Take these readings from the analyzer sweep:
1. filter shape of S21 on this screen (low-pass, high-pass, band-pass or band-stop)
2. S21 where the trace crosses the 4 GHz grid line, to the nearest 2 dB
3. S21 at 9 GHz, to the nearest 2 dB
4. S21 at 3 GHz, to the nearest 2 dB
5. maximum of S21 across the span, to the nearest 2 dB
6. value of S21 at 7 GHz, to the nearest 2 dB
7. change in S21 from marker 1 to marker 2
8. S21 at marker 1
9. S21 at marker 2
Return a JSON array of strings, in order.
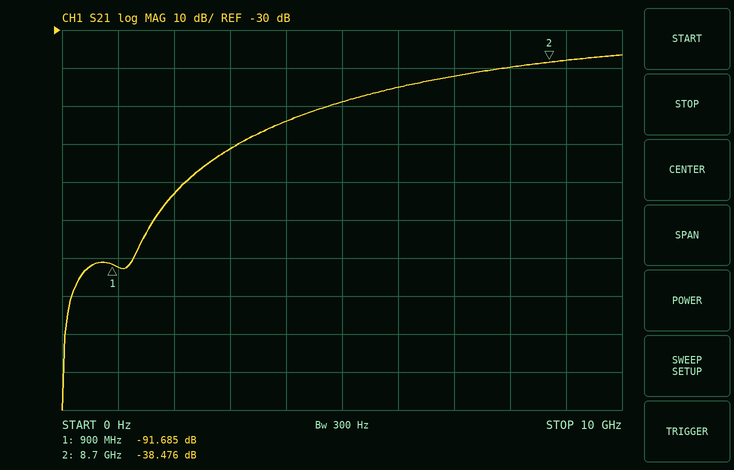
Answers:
["high-pass", "-54 dB", "-38 dB", "-62 dB", "-36 dB", "-42 dB", "53.209 dB", "-91.685 dB", "-38.476 dB"]
